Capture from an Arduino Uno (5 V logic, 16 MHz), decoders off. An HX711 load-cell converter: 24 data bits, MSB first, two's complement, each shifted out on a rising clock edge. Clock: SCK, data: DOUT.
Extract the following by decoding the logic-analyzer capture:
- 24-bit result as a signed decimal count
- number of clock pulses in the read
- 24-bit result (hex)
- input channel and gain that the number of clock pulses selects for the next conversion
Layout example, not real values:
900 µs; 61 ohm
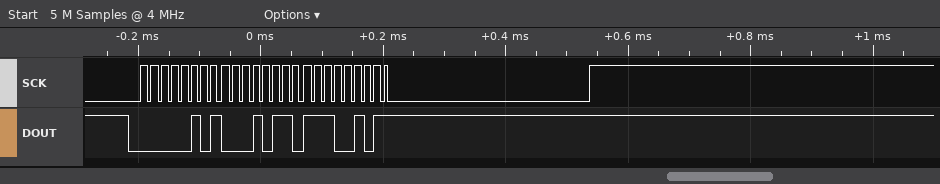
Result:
333541; 26; 0x0516E5; channel B, gain 32
